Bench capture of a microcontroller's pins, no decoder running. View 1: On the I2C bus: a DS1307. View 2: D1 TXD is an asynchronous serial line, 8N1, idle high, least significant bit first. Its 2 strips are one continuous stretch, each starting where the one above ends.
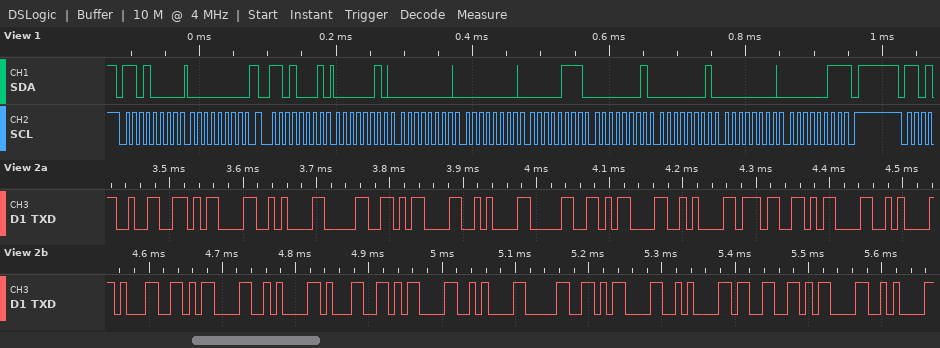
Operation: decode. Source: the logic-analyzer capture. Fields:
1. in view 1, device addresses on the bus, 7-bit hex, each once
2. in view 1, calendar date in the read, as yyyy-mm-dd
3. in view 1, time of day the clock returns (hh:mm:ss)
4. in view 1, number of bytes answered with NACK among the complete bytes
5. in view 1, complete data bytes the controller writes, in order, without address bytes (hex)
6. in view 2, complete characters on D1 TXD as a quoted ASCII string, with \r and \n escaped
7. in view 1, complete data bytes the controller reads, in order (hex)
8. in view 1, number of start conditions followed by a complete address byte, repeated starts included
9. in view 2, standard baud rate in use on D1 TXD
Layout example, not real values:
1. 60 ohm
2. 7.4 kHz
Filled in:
1. 0x68
2. 2000-01-01
3. 00:00:02
4. 1
5. 00
6. "2\r\n0\r\n0\r\n7\r\n1\r\n1\r\n0\r\n3\r\n"
7. 02 00 00 07 01 01 00 03
8. 2
9. 115200 baud
